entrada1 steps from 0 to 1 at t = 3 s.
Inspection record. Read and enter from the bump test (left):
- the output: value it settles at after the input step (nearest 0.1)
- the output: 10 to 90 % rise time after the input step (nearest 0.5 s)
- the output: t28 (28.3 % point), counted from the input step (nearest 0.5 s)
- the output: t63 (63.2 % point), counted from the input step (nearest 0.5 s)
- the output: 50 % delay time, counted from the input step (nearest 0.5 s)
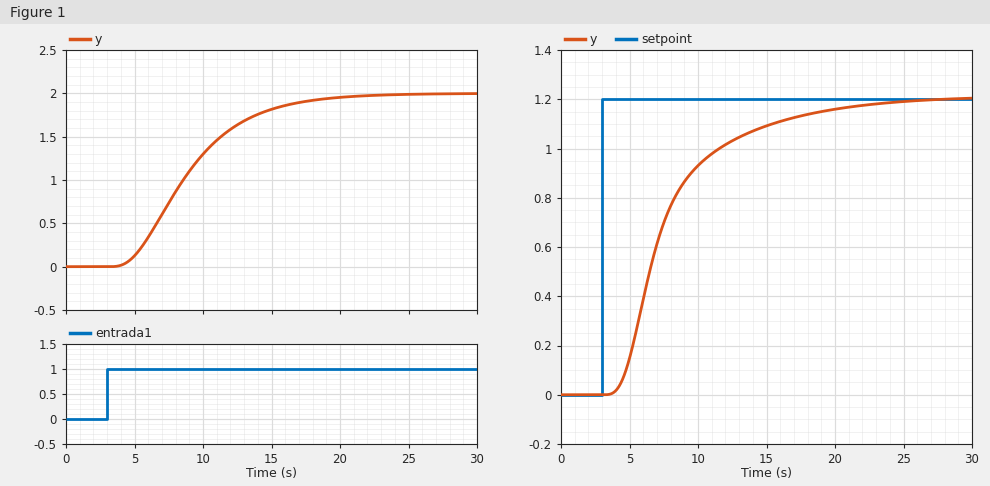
2.0
9.5 s
4.0 s
7.0 s
5.5 s
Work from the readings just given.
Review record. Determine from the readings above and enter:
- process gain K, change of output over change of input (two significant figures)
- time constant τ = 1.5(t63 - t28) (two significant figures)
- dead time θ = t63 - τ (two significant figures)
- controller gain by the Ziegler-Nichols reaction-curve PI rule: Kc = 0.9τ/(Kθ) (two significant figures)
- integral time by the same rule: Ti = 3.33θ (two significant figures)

2.0
4.5 s
2.5 s
0.81
8.3 s
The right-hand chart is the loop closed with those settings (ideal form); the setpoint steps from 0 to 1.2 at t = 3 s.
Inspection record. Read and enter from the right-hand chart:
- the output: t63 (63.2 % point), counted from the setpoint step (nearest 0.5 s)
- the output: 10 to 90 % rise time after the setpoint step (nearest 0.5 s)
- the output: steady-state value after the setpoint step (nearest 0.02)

5.0 s
9.5 s
1.20
